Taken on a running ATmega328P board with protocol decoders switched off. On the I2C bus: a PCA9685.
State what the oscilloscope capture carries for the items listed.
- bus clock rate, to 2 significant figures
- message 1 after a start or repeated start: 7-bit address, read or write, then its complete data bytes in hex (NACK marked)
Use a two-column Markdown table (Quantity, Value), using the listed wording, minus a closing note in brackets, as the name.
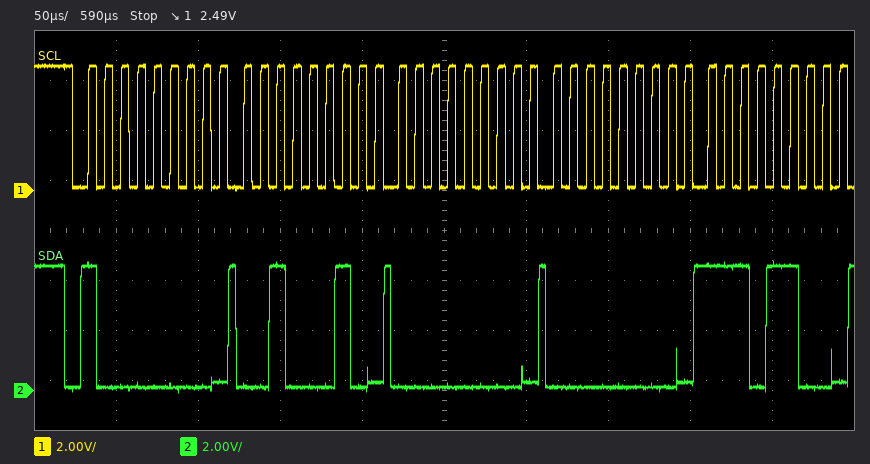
| Quantity | Value |
|---|---|
| bus clock rate, to 2 significant figures | 100 kHz |
| message 1 after a start or repeated start: 7-bit address, read or write, then its complete data bytes in hex | 0x40 write: 22 00 00 EC |
